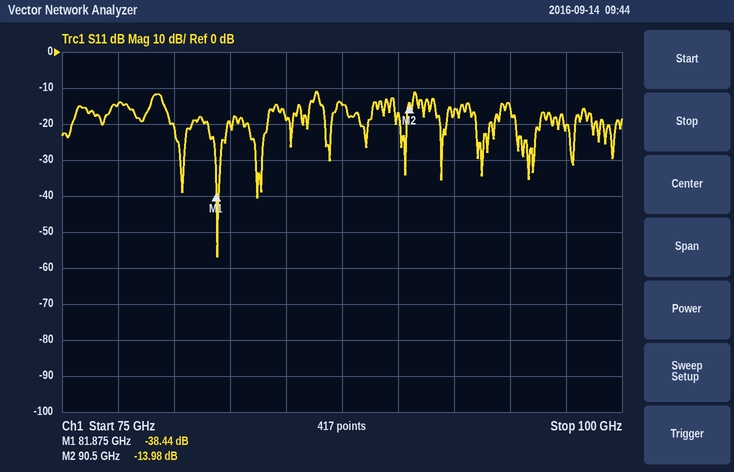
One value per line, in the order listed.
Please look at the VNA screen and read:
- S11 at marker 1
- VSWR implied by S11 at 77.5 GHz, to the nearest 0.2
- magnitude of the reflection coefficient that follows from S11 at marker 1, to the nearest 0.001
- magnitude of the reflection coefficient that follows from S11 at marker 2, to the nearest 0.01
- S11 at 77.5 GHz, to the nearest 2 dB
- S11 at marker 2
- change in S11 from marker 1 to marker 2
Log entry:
-38.44 dB
1.4
0.012
0.20
-14 dB
-13.98 dB
24.46 dB
